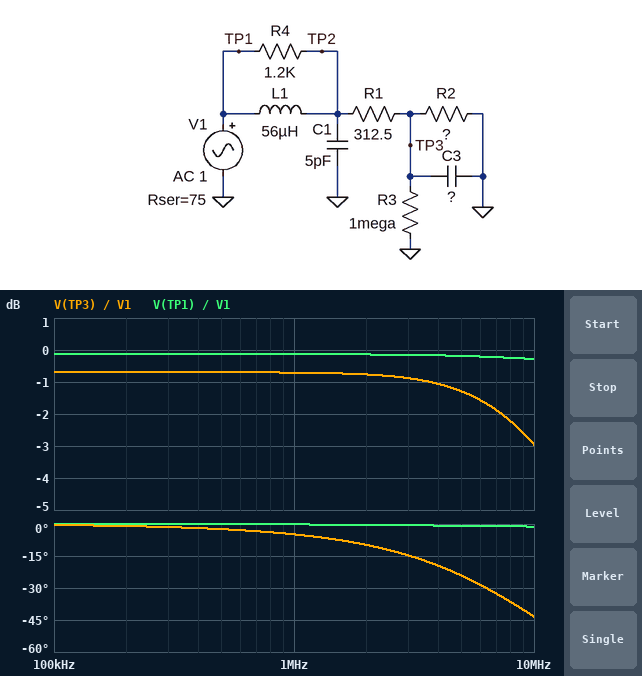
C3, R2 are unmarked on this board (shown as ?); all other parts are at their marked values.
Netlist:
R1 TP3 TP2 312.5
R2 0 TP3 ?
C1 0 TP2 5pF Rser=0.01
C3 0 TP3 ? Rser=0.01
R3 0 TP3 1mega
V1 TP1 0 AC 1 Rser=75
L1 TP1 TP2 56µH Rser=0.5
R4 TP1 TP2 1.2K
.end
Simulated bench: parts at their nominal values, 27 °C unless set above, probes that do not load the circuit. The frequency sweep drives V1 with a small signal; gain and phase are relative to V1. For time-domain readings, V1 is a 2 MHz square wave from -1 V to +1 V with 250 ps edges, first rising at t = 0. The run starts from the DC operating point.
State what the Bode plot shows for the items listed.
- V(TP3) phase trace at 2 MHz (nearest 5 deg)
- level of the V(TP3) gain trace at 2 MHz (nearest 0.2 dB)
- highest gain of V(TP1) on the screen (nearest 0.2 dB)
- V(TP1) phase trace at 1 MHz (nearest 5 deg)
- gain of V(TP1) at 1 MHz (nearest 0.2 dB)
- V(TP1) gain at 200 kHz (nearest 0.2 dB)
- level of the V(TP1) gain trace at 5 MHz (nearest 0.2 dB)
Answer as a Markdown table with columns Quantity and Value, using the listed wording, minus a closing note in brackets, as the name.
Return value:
| Quantity | Value |
|---|---|
| V(TP3) phase trace at 2 MHz | -10 deg |
| level of the V(TP3) gain trace at 2 MHz | -0.8 dB |
| highest gain of V(TP1) on the screen | -0.2 dB |
| V(TP1) phase trace at 1 MHz | 0 deg |
| gain of V(TP1) at 1 MHz | -0.2 dB |
| V(TP1) gain at 200 kHz | -0.2 dB |
| level of the V(TP1) gain trace at 5 MHz | -0.2 dB |
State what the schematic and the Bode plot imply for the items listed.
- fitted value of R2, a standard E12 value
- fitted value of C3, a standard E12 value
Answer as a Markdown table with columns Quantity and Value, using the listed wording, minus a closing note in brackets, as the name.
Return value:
| Quantity | Value |
|---|---|
| fitted value of R2, a standard E12 value | 4.7 kΩ |
| fitted value of C3, a standard E12 value | 5.6 pF |
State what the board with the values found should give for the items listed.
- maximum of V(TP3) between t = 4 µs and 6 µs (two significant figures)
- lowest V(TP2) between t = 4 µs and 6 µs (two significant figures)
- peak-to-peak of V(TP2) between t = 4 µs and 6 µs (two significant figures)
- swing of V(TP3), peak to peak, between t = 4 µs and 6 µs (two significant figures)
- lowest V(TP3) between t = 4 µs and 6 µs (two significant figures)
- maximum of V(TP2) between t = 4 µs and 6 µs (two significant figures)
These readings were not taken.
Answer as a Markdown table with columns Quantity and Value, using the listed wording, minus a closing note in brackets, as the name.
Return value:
| Quantity | Value |
|---|---|
| maximum of V(TP3) between t = 4 µs and 6 µs | 930 mV |
| lowest V(TP2) between t = 4 µs and 6 µs | -990 mV |
| peak-to-peak of V(TP2) between t = 4 µs and 6 µs | 2.0 V |
| swing of V(TP3), peak to peak, between t = 4 µs and 6 µs | 1.9 V |
| lowest V(TP3) between t = 4 µs and 6 µs | -930 mV |
| maximum of V(TP2) between t = 4 µs and 6 µs | 990 mV |
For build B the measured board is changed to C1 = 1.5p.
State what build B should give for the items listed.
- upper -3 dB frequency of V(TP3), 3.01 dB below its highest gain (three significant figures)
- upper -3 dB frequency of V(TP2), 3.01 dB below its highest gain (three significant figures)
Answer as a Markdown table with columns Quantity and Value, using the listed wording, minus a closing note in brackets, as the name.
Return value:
| Quantity | Value |
|---|---|
| upper -3 dB frequency of V(TP3), 3.01 dB below its highest gain | 15.0 MHz |
| upper -3 dB frequency of V(TP2), 3.01 dB below its highest gain | 15.5 MHz |
